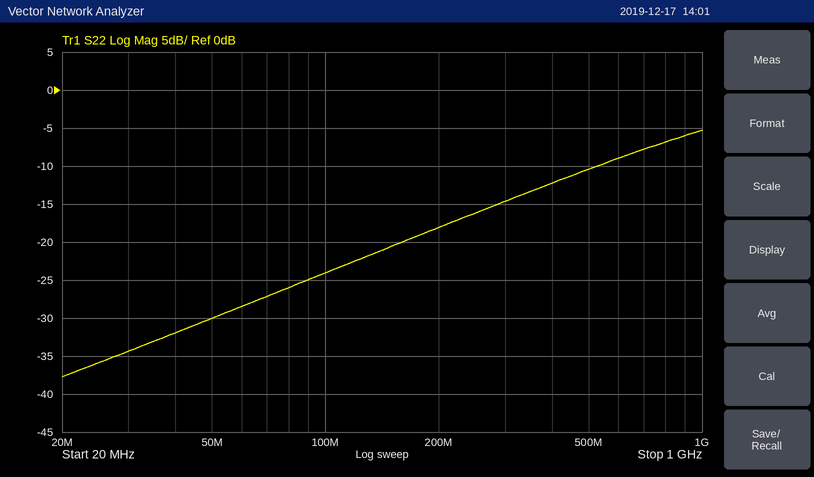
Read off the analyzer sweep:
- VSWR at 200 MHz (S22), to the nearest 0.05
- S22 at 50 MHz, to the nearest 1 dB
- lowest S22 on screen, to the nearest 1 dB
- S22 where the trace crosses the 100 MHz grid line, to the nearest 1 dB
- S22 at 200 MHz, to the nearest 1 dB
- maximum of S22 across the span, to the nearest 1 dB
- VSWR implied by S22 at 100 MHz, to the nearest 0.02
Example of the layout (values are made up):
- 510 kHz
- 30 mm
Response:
- 1.30
- -30 dB
- -38 dB
- -24 dB
- -18 dB
- -5 dB
- 1.14
